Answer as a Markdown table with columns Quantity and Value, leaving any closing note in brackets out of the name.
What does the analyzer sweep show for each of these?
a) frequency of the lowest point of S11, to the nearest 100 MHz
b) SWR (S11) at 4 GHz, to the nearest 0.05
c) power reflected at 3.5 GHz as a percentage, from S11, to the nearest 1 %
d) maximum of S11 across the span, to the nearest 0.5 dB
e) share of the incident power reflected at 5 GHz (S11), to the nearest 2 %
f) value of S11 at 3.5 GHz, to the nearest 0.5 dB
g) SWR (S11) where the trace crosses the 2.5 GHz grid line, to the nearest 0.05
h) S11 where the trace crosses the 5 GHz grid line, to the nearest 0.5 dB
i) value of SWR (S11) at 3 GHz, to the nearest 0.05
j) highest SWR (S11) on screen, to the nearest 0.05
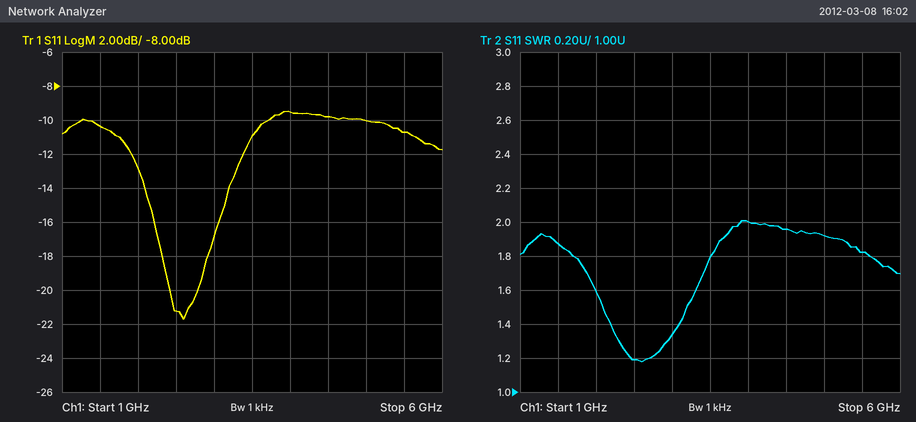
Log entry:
| Quantity | Value |
|---|---|
| frequency of the lowest point of S11, to the nearest 100 MHz | 2.6 GHz |
| SWR (S11) at 4 GHz, to the nearest 0.05 | 2.00 |
| power reflected at 3.5 GHz as a percentage, from S11, to the nearest 1 % | 8 % |
| maximum of S11 across the span, to the nearest 0.5 dB | -9.5 dB |
| share of the incident power reflected at 5 GHz (S11), to the nearest 2 % | 10 % |
| value of S11 at 3.5 GHz, to the nearest 0.5 dB | -11.0 dB |
| SWR (S11) where the trace crosses the 2.5 GHz grid line, to the nearest 0.05 | 1.20 |
| S11 where the trace crosses the 5 GHz grid line, to the nearest 0.5 dB | -10.0 dB |
| value of SWR (S11) at 3 GHz, to the nearest 0.05 | 1.35 |
| highest SWR (S11) on screen, to the nearest 0.05 | 2.00 |
